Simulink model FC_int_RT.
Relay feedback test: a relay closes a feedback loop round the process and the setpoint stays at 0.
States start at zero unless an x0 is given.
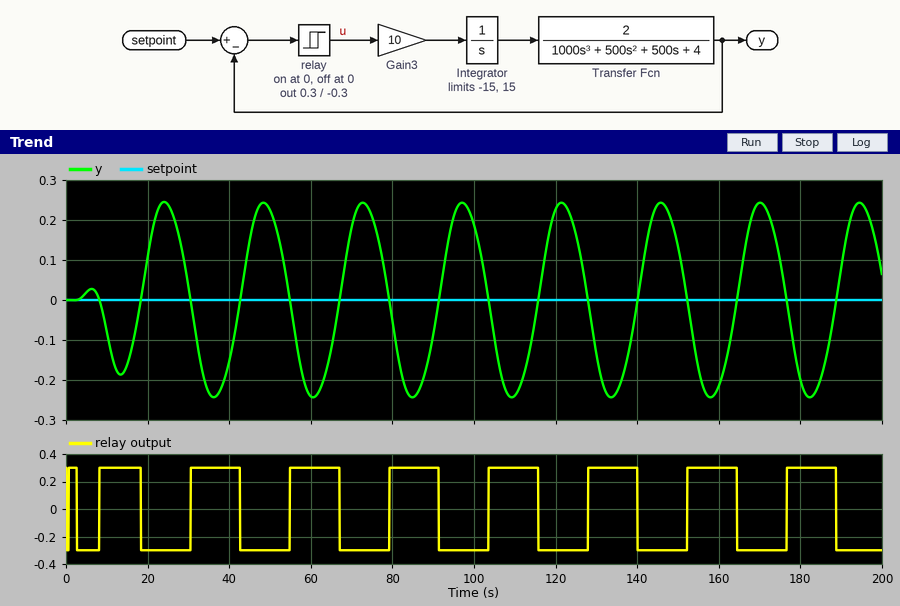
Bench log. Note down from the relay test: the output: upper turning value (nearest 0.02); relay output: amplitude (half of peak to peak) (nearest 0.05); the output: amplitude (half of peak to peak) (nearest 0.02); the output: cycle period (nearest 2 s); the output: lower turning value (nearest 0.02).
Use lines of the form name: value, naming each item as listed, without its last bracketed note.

the output: upper turning value: 0.24
relay output: amplitude (half of peak to peak): 0.30
the output: amplitude (half of peak to peak): 0.24
the output: cycle period: 24 s
the output: lower turning value: -0.24
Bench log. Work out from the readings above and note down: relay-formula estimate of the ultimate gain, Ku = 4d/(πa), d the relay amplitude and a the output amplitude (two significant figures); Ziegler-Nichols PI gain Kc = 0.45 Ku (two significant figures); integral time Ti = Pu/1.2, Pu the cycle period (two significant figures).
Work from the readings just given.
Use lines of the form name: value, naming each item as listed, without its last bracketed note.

relay-formula estimate of the ultimate gain, Ku = 4d/(πa), d the relay amplitude and a the output amplitude: 1.6
Ziegler-Nichols PI gain Kc = 0.45 Ku: 0.72
integral time Ti = Pu/1.2, Pu the cycle period: 20 s
